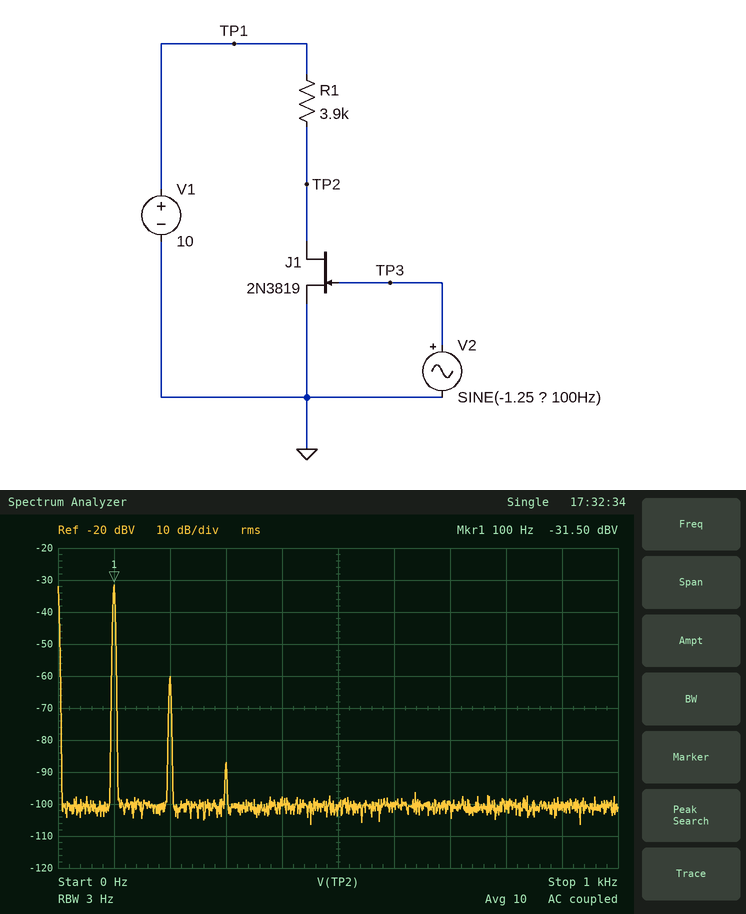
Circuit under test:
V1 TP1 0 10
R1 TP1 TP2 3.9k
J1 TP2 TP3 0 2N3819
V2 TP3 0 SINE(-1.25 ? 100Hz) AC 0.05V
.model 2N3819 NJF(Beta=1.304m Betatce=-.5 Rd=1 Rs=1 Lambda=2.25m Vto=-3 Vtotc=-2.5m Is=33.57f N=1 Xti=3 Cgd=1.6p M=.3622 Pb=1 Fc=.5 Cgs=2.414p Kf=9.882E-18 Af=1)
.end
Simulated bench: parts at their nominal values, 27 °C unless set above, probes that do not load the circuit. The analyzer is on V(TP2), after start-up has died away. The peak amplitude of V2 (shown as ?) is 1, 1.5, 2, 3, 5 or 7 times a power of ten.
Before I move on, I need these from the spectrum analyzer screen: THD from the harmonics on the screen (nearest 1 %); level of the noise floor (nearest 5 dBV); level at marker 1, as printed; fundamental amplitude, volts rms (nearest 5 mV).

4 %
-100 dBV
-31.50 dBV
25 mV
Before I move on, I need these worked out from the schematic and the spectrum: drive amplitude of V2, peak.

70 mV
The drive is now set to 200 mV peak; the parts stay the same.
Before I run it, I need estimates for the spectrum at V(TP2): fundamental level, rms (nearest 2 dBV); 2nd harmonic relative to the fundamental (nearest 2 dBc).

-22 dBV
-20 dBc
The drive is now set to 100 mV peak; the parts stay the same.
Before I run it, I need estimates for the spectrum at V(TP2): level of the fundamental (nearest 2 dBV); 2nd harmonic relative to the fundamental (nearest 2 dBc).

-28 dBV
-26 dBc
